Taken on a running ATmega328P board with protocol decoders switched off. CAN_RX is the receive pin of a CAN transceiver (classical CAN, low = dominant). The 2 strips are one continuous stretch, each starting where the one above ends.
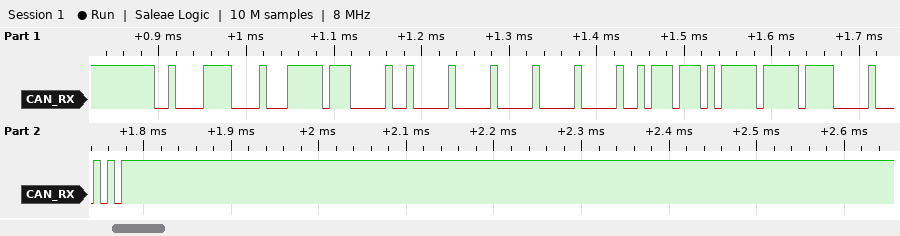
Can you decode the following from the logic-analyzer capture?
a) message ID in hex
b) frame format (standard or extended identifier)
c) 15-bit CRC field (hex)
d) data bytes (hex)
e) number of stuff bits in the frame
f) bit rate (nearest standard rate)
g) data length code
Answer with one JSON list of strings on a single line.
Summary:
["0x21E", "standard", "0x7C02", "FF 01 00 00 00 17 75 FF", "10", "125 kbit/s", "8"]
